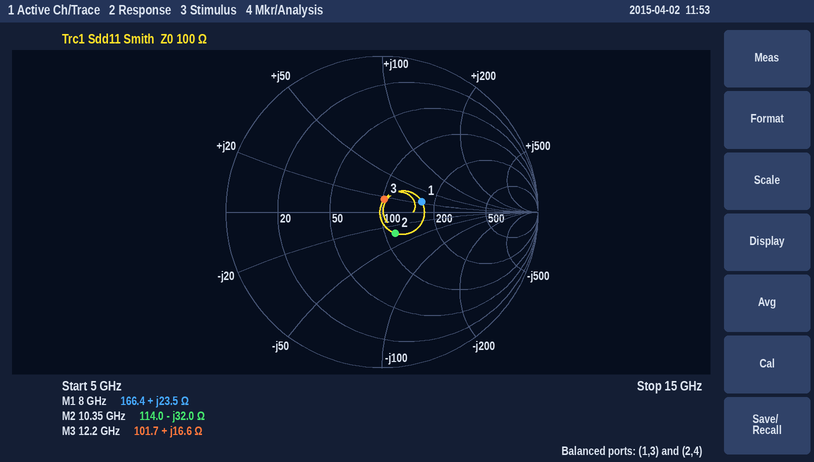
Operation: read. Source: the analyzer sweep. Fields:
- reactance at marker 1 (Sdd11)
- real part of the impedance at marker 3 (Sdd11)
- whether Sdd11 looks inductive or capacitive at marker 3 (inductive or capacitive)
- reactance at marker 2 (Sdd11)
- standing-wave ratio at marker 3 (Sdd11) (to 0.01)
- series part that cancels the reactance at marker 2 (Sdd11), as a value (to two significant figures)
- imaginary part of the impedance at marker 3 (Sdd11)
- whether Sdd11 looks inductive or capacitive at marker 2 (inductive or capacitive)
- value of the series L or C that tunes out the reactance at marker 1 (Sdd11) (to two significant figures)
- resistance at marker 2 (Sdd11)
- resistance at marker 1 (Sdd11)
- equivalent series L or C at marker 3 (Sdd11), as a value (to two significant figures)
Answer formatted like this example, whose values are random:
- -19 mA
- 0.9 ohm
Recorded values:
- +23.5 Ω
- 101.7 Ω
- inductive
- -32.0 Ω
- 1.18
- 490 pH
- +16.6 Ω
- capacitive
- 850 fF
- 114.0 Ω
- 166.4 Ω
- 220 pH
